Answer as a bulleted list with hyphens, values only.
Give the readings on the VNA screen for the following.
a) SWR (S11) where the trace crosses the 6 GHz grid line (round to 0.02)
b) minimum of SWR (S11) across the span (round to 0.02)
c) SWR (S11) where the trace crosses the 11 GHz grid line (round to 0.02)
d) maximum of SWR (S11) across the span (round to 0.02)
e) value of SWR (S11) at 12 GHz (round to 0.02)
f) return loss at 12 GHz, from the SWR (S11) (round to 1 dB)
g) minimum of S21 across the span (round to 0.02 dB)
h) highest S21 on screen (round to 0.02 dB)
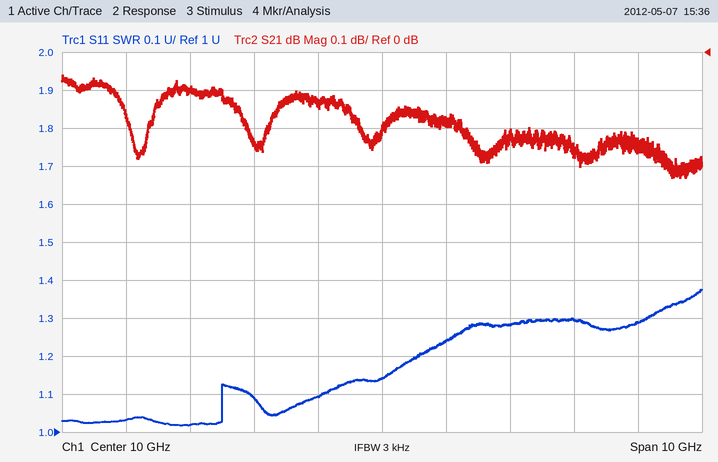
- 1.04
- 1.02
- 1.24
- 1.38
- 1.28
- 18 dB
- -0.34 dB
- -0.06 dB
